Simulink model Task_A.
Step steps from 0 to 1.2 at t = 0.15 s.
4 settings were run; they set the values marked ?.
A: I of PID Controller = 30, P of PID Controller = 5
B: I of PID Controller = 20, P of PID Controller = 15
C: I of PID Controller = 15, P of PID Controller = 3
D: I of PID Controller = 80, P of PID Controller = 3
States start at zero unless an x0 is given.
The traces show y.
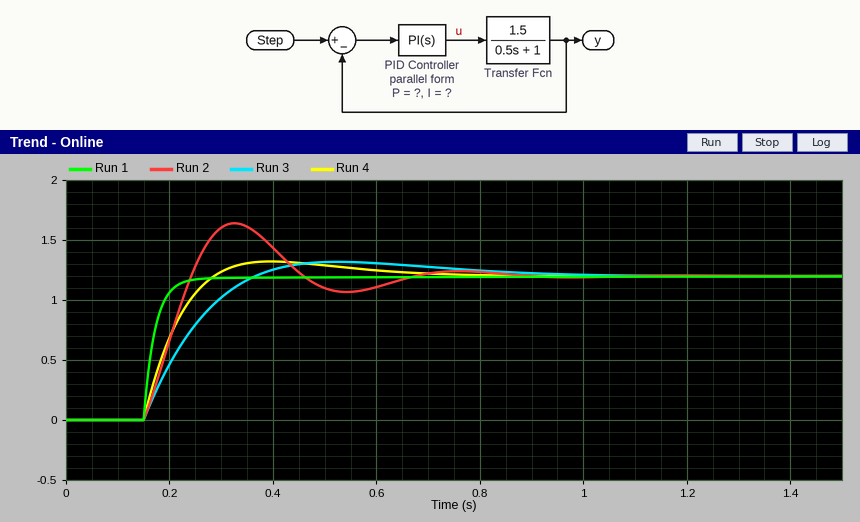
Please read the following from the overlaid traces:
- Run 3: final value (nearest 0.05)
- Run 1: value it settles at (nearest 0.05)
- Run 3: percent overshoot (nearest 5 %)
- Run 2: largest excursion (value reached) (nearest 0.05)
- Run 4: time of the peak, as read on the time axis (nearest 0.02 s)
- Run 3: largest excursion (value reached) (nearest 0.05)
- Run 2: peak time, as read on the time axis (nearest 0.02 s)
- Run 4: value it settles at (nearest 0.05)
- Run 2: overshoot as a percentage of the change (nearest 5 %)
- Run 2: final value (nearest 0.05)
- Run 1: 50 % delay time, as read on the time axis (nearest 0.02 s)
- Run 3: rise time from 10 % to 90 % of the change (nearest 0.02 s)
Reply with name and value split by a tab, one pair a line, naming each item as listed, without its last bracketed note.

Run 3: final value	1.20
Run 1: value it settles at	1.20
Run 3: percent overshoot	10 %
Run 2: largest excursion (value reached)	1.65
Run 4: time of the peak, as read on the time axis	0.40 s
Run 3: largest excursion (value reached)	1.30
Run 2: peak time, as read on the time axis	0.32 s
Run 4: value it settles at	1.20
Run 2: overshoot as a percentage of the change	35 %
Run 2: final value	1.20
Run 1: 50 % delay time, as read on the time axis	0.16 s
Run 3: rise time from 10 % to 90 % of the change	0.16 s
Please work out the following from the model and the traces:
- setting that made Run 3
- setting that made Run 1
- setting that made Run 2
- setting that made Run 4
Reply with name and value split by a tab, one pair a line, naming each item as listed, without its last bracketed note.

setting that made Run 3	C
setting that made Run 1	B
setting that made Run 2	D
setting that made Run 4	A
